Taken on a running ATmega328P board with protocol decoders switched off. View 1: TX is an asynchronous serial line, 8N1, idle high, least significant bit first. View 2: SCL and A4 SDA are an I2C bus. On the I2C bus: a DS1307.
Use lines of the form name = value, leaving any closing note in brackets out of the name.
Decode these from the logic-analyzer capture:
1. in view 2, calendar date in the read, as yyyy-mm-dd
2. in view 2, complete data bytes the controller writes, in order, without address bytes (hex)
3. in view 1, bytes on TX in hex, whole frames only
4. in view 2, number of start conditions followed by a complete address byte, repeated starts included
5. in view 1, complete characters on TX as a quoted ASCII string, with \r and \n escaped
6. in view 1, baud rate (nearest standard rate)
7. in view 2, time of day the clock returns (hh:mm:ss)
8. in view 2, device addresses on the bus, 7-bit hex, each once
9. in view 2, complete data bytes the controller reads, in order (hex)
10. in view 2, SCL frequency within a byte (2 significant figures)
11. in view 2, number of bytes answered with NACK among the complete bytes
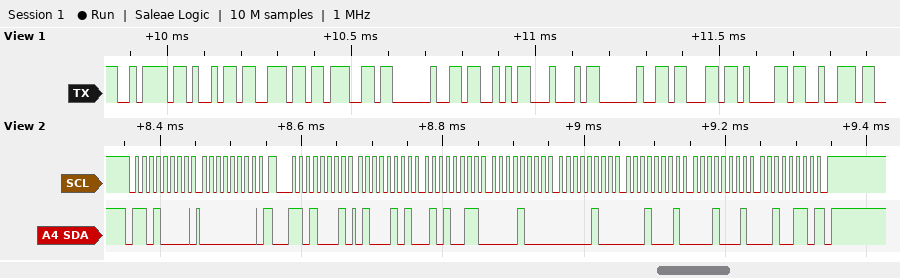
in view 2, calendar date in the read, as yyyy-mm-dd = 2026-11-11
in view 2, complete data bytes the controller writes, in order, without address bytes = 00
in view 1, bytes on TX in hex, whole frames only = 7A 69 6E 67 20 53 44 20 63 61 72
in view 2, number of start conditions followed by a complete address byte, repeated starts included = 2
in view 1, complete characters on TX as a quoted ASCII string, with \r and \n escaped = "zing SD car"
in view 1, baud rate = 57600 baud
in view 2, time of day the clock returns = 08:53:45
in view 2, device addresses on the bus, 7-bit hex, each once = 0x68
in view 2, complete data bytes the controller reads, in order = 45 53 08 04 11 11 26
in view 2, SCL frequency within a byte = 100 kHz
in view 2, number of bytes answered with NACK among the complete bytes = 1
